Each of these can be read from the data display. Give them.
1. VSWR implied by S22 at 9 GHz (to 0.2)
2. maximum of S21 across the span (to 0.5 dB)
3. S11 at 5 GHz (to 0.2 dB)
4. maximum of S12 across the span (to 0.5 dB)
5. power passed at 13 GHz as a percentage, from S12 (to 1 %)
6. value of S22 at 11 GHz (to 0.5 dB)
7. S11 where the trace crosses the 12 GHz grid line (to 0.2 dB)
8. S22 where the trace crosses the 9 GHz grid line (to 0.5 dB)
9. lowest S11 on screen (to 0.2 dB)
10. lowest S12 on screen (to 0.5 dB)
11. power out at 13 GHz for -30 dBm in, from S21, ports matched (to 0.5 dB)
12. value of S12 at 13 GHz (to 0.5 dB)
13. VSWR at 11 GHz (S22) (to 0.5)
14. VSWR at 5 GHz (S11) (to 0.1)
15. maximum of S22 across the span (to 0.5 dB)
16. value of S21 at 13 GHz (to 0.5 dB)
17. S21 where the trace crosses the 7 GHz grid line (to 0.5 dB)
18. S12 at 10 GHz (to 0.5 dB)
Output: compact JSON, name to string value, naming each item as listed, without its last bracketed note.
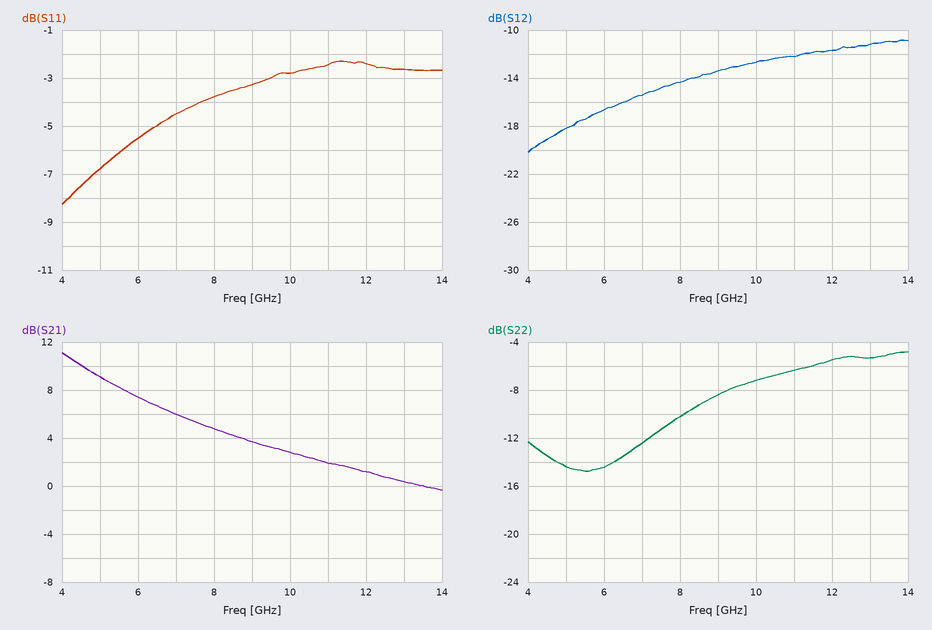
{"VSWR implied by S22 at 9 GHz": "2.2", "maximum of S21 across the span": "11.0 dB", "S11 at 5 GHz": "-6.8 dB", "maximum of S12 across the span": "-11.0 dB", "power passed at 13 GHz as a percentage, from S12": "8 %", "value of S22 at 11 GHz": "-6.5 dB", "S11 where the trace crosses the 12 GHz grid line": "-2.4 dB", "S22 where the trace crosses the 9 GHz grid line": "-8.5 dB", "lowest S11 on screen": "-8.2 dB", "lowest S12 on screen": "-20.0 dB", "power out at 13 GHz for -30 dBm in, from S21, ports matched": "-29.5 dBm", "value of S12 at 13 GHz": "-11.0 dB", "VSWR at 11 GHz (S22)": "3.0", "VSWR at 5 GHz (S11)": "2.7", "maximum of S22 across the span": "-5.0 dB", "value of S21 at 13 GHz": "0.5 dB", "S21 where the trace crosses the 7 GHz grid line": "6.0 dB", "S12 at 10 GHz": "-12.5 dB"}
